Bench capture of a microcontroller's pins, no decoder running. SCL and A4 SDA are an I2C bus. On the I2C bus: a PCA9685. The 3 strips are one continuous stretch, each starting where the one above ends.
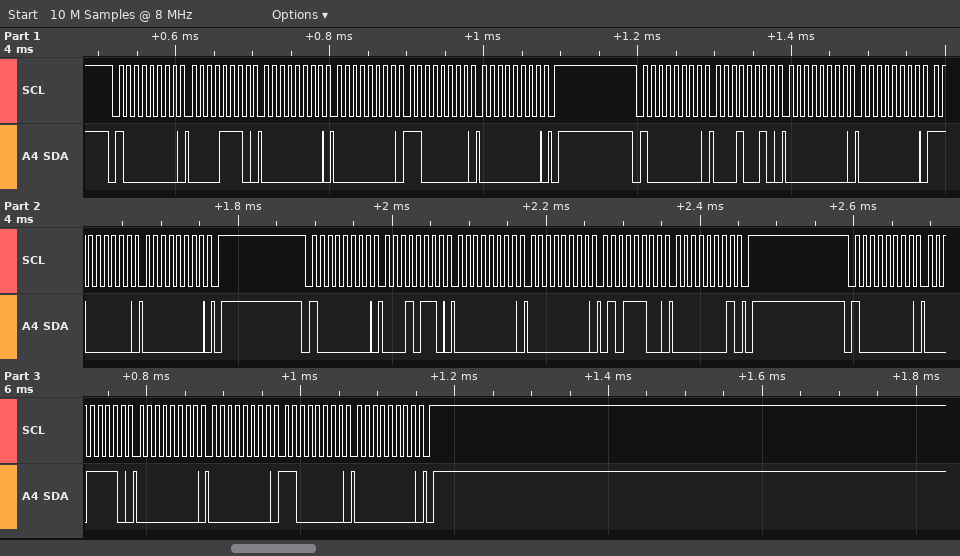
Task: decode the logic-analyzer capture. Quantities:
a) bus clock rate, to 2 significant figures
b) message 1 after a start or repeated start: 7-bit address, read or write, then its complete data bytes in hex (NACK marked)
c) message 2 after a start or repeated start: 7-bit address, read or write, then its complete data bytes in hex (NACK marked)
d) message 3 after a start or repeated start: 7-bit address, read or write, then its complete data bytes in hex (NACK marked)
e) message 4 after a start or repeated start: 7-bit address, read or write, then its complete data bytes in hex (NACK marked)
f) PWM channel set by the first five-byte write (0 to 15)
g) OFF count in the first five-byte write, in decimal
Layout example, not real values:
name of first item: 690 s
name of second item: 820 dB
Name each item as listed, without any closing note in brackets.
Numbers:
bus clock rate, to 2 significant figures: 100 kHz
message 1 after a start or repeated start: 7-bit address, read or write, then its complete data bytes in hex: 0x40 write: 0E 00 00 C0 00
message 2 after a start or repeated start: 7-bit address, read or write, then its complete data bytes in hex: 0x40 write: 12 00 00 C0 00
message 3 after a start or repeated start: 7-bit address, read or write, then its complete data bytes in hex: 0x40 write: 16 00 00 5C 01
message 4 after a start or repeated start: 7-bit address, read or write, then its complete data bytes in hex: 0x40 write: 1E 00 00 C0 00
PWM channel set by the first five-byte write: 2
OFF count in the first five-byte write, in decimal: 192
